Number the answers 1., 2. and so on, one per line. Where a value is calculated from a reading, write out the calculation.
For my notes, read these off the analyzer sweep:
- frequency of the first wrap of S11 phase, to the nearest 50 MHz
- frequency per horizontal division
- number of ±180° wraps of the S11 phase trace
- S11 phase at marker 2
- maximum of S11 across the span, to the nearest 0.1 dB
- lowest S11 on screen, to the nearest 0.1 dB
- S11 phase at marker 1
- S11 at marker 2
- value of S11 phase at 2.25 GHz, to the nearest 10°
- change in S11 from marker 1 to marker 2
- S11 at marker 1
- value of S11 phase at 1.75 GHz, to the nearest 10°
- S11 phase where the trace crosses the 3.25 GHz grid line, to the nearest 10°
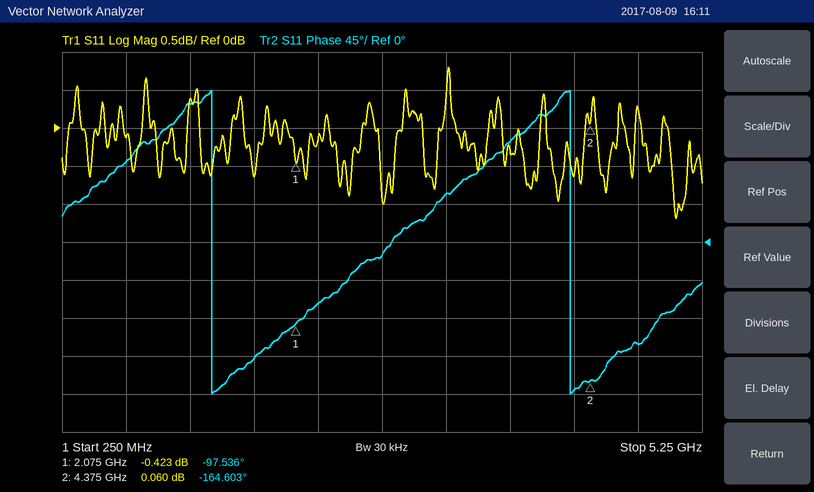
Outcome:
1. 1.40 GHz
2. 500 MHz
3. 2
4. -164.603°
5. 0.8 dB
6. -1.2 dB
7. -97.536°
8. 0.060 dB
9. -70°
10. 0.06 − (-0.423) = 0.483 dB
11. -0.423 dB
12. -140°
13. 60°
